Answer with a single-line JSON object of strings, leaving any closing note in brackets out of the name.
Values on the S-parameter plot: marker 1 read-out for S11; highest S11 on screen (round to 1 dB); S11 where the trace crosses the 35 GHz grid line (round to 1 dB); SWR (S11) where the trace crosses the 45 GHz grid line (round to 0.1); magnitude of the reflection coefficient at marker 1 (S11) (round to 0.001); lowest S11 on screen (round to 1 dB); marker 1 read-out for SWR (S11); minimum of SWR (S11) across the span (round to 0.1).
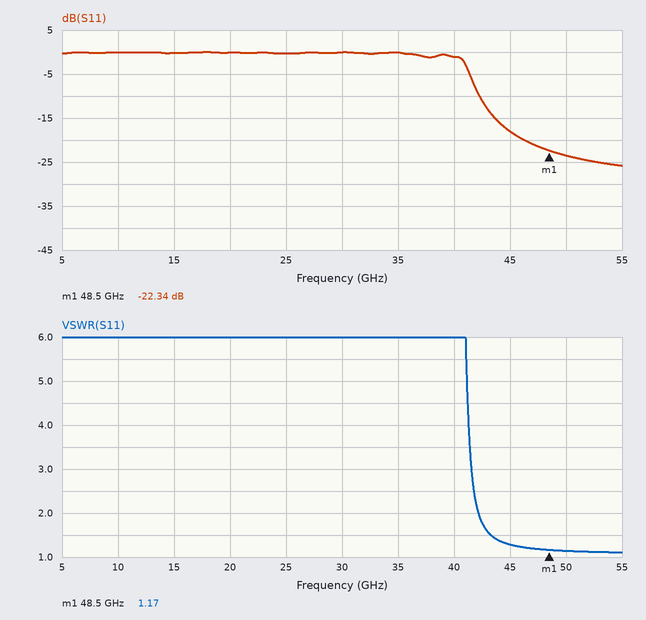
{"marker 1 read-out for S11": "-22.34 dB", "highest S11 on screen": "0 dB", "S11 where the trace crosses the 35 GHz grid line": "0 dB", "SWR (S11) where the trace crosses the 45 GHz grid line": "1.3", "magnitude of the reflection coefficient at marker 1 (S11)": "0.076", "lowest S11 on screen": "-26 dB", "marker 1 read-out for SWR": "1.17", "minimum of SWR (S11) across the span": "1.1"}
